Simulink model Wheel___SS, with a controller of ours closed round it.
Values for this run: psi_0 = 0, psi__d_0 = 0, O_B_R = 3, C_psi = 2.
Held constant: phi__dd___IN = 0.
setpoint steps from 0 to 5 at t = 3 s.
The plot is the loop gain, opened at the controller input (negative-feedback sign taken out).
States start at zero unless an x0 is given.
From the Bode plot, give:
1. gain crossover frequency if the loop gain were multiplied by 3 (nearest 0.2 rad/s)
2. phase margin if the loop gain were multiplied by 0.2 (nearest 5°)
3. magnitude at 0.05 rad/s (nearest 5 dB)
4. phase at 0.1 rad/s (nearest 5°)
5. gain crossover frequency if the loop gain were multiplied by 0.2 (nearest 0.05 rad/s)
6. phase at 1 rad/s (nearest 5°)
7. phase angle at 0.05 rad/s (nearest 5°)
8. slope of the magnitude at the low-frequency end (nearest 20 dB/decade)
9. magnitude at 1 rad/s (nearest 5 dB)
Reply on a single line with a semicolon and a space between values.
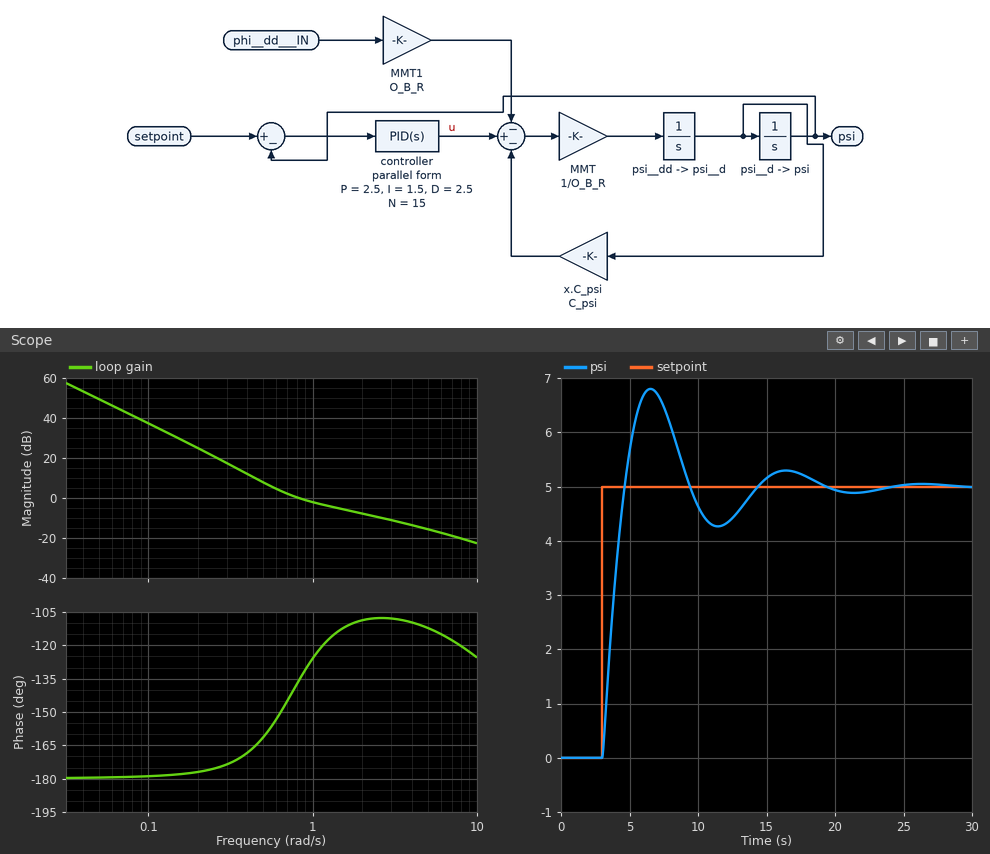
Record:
2.6 rad/s; 10°; 50 dB; -180°; 0.35 rad/s; -125°; -180°; -40 dB/decade; 0 dB
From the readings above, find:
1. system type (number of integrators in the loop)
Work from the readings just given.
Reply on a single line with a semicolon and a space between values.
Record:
2
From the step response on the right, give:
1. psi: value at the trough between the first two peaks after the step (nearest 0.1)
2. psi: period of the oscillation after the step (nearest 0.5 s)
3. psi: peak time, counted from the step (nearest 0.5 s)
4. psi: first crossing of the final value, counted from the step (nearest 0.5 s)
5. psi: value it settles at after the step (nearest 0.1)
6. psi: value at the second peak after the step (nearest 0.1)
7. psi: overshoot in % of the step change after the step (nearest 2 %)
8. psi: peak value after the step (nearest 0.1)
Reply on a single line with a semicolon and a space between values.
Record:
4.3; 10.0 s; 3.5 s; 1.5 s; 5.0; 5.3; 36 %; 6.8
